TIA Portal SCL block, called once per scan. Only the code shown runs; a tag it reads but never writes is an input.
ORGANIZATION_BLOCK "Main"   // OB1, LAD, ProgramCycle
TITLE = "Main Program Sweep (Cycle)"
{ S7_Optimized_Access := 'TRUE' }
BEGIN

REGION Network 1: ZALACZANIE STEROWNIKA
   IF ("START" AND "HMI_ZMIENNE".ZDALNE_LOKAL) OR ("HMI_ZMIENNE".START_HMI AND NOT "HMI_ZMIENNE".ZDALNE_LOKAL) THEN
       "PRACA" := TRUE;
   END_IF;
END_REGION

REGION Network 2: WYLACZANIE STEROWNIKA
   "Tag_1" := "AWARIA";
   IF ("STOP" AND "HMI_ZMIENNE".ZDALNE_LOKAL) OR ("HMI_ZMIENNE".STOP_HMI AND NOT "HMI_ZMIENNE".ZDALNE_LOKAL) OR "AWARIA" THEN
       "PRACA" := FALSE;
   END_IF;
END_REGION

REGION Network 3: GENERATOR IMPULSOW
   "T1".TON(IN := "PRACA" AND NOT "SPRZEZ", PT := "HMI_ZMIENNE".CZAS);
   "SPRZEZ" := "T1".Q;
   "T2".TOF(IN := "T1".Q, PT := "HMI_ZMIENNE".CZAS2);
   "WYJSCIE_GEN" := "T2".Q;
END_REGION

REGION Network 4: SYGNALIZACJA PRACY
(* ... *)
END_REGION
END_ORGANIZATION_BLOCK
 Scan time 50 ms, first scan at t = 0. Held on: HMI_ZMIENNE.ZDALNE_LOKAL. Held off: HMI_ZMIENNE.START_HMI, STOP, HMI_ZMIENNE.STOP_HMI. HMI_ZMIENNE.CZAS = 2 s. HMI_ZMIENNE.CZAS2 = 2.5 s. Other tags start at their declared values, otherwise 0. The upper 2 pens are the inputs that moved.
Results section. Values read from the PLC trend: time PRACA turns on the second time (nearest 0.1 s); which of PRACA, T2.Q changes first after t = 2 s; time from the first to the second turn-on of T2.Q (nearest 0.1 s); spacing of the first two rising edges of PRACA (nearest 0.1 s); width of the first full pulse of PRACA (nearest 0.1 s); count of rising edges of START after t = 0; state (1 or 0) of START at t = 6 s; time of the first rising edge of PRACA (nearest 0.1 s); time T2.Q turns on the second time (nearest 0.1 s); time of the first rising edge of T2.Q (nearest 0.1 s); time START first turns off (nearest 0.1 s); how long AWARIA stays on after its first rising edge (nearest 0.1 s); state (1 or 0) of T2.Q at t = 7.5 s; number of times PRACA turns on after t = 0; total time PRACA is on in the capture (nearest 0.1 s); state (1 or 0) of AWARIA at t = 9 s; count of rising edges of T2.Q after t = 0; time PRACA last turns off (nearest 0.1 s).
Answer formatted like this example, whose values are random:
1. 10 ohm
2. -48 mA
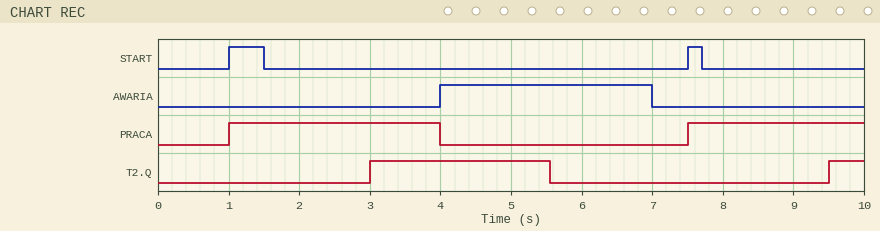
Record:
1. 7.5 s
2. T2.Q
3. 6.5 s
4. 6.5 s
5. 3.0 s
6. 2
7. 0
8. 1.0 s
9. 9.5 s
10. 3.0 s
11. 1.5 s
12. 3.0 s
13. 0
14. 2
15. 5.5 s
16. 0
17. 2
18. 4.0 s
